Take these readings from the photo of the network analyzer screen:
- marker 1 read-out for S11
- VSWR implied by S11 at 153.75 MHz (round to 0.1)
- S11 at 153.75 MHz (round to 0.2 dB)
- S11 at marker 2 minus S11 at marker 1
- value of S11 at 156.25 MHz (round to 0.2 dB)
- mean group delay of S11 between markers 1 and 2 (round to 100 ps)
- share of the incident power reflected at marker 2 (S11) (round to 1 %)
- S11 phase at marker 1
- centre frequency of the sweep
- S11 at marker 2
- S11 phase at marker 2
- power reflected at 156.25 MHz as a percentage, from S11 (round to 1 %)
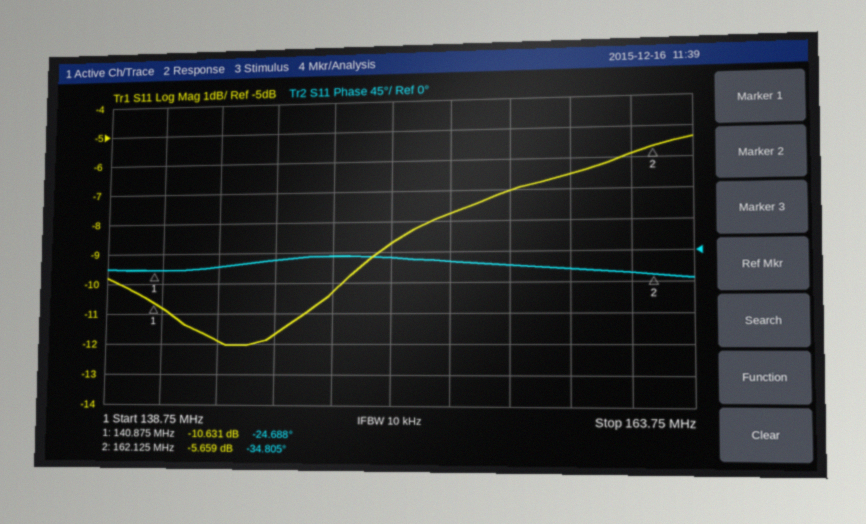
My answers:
-10.631 dB
2.4
-7.8 dB
4.972 dB
-7.0 dB
1.3 ns
27 %
-24.688°
151.25 MHz
-5.659 dB
-34.805°
20 %
